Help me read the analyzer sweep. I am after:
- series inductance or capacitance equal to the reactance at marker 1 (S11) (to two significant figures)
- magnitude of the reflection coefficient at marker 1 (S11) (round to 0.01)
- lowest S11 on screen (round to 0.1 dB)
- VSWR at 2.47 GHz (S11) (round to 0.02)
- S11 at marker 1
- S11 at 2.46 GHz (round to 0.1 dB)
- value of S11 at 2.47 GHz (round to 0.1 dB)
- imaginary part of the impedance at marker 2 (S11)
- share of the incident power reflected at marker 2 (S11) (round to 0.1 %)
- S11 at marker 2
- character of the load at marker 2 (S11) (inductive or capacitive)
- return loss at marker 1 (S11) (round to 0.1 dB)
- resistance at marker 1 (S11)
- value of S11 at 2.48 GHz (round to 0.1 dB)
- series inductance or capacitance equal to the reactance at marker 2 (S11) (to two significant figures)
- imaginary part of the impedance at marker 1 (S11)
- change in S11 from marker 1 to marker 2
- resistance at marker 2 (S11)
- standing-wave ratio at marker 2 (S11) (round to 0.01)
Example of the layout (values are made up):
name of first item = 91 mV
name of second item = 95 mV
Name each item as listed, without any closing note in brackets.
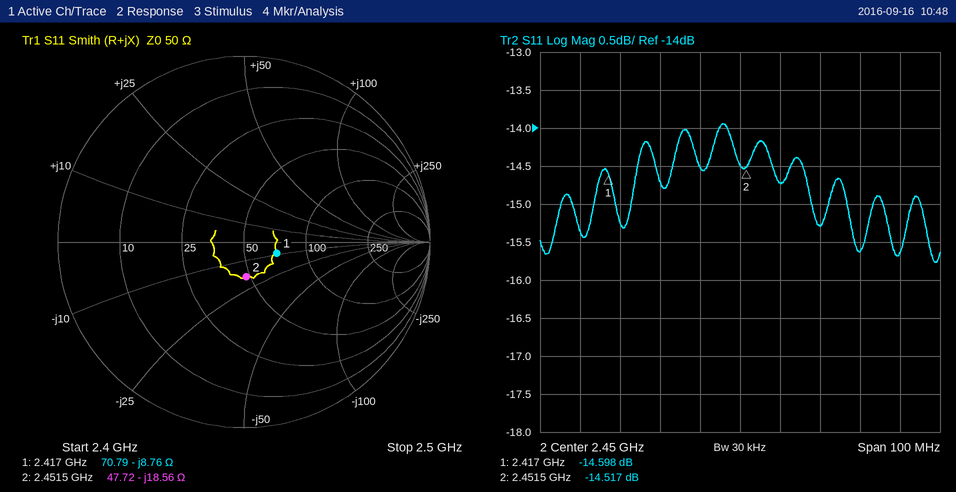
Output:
series inductance or capacitance equal to the reactance at marker 1 (S11) = 7.5 pF
magnitude of the reflection coefficient at marker 1 (S11) = 0.19
lowest S11 on screen = -15.8 dB
VSWR at 2.47 GHz (S11) = 1.42
S11 at marker 1 = -14.598 dB
S11 at 2.46 GHz = -14.7 dB
value of S11 at 2.47 GHz = -15.3 dB
imaginary part of the impedance at marker 2 = -18.56 Ω
share of the incident power reflected at marker 2 (S11) = 3.5 %
S11 at marker 2 = -14.517 dB
character of the load at marker 2 (S11) = capacitive
return loss at marker 1 (S11) = 14.6 dB
resistance at marker 1 = 70.79 Ω
value of S11 at 2.48 GHz = -15.6 dB
series inductance or capacitance equal to the reactance at marker 2 (S11) = 3.5 pF
imaginary part of the impedance at marker 1 = -8.76 Ω
change in S11 from marker 1 to marker 2 = 0.081 dB
resistance at marker 2 = 47.72 Ω
standing-wave ratio at marker 2 (S11) = 1.46
